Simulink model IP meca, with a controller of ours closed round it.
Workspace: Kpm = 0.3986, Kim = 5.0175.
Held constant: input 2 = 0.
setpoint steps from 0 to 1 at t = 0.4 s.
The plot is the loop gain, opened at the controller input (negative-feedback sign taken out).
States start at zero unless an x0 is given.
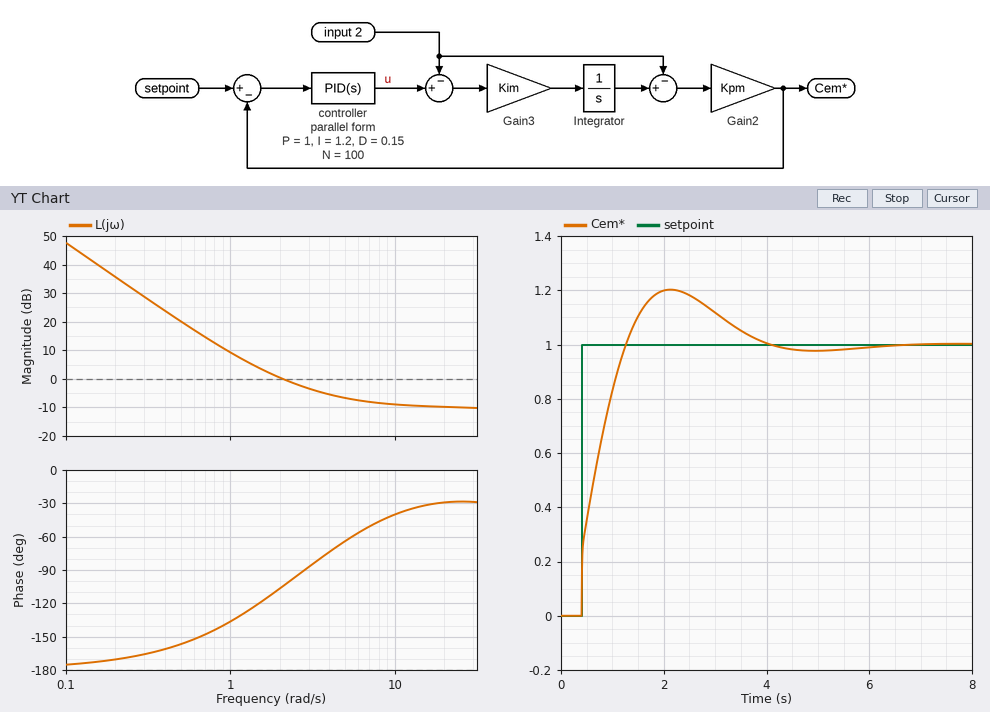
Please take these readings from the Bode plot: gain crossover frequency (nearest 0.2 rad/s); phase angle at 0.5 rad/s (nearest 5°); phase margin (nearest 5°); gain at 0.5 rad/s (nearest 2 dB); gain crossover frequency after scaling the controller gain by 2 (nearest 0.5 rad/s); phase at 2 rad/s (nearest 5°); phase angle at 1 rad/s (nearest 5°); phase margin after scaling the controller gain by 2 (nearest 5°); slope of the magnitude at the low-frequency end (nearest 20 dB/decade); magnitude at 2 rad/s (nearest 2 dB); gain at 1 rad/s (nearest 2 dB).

2.0 rad/s
-155°
75°
20 dB
4.5 rad/s
-105°
-135°
110°
-40 dB/decade
0 dB
10 dB
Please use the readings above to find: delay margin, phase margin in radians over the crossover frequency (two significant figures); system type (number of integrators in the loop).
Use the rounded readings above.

0.65 s
2
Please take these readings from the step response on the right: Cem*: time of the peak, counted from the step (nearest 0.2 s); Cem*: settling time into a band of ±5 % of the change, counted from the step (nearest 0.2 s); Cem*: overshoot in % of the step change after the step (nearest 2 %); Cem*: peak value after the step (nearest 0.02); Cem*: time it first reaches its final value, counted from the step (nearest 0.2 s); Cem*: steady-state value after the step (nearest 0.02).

1.8 s
3.2 s
20 %
1.20
0.8 s
1.00
